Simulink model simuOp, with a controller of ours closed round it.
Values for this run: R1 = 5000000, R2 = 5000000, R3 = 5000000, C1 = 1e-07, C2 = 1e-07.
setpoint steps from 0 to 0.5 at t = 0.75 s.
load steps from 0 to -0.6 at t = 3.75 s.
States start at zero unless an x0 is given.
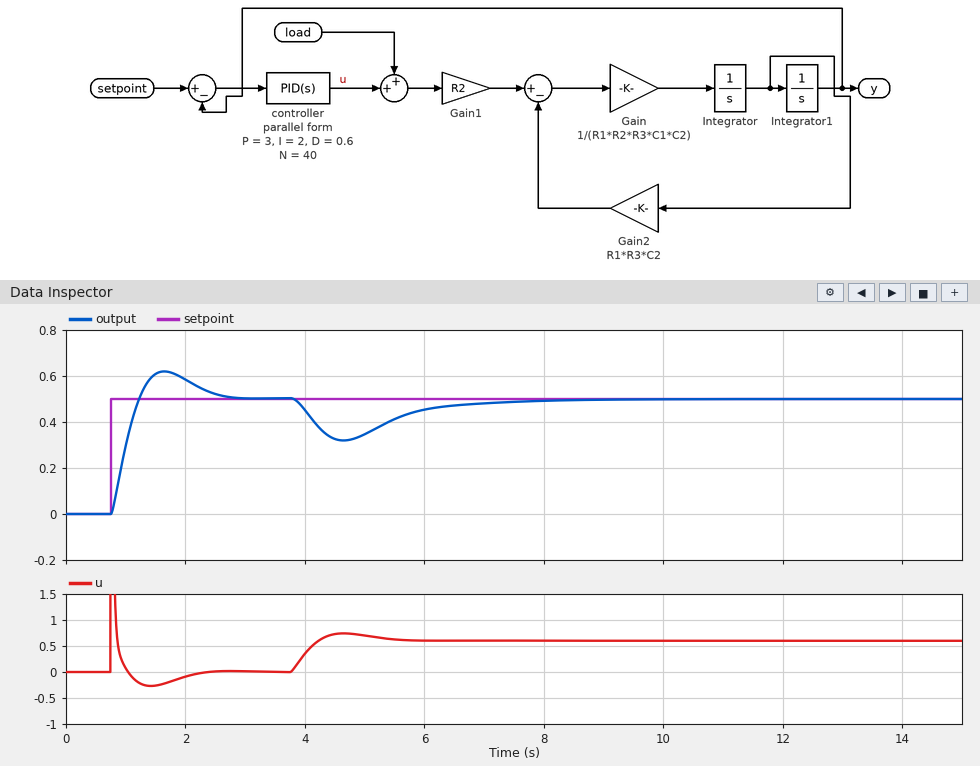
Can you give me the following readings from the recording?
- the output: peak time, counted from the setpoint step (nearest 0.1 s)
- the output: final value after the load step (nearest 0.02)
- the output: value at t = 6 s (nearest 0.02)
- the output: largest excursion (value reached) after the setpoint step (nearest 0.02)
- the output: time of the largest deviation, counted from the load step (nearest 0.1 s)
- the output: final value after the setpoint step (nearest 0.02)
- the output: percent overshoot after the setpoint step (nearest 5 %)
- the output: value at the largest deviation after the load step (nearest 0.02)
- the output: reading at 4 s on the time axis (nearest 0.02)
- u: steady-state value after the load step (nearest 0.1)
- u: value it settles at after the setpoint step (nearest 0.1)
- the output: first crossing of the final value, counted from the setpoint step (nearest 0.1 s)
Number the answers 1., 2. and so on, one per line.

1. 0.9 s
2. 0.50
3. 0.46
4. 0.62
5. 0.9 s
6. 0.50
7. 25 %
8. 0.32
9. 0.46
10. 0.6
11. 0.0
12. 0.5 s
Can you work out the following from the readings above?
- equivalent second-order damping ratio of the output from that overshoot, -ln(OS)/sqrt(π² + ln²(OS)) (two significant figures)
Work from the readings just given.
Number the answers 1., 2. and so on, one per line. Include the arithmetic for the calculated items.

1. ln(0.25) = -1.386; 1.386 / sqrt(9.870 + 1.922) = 0.40
